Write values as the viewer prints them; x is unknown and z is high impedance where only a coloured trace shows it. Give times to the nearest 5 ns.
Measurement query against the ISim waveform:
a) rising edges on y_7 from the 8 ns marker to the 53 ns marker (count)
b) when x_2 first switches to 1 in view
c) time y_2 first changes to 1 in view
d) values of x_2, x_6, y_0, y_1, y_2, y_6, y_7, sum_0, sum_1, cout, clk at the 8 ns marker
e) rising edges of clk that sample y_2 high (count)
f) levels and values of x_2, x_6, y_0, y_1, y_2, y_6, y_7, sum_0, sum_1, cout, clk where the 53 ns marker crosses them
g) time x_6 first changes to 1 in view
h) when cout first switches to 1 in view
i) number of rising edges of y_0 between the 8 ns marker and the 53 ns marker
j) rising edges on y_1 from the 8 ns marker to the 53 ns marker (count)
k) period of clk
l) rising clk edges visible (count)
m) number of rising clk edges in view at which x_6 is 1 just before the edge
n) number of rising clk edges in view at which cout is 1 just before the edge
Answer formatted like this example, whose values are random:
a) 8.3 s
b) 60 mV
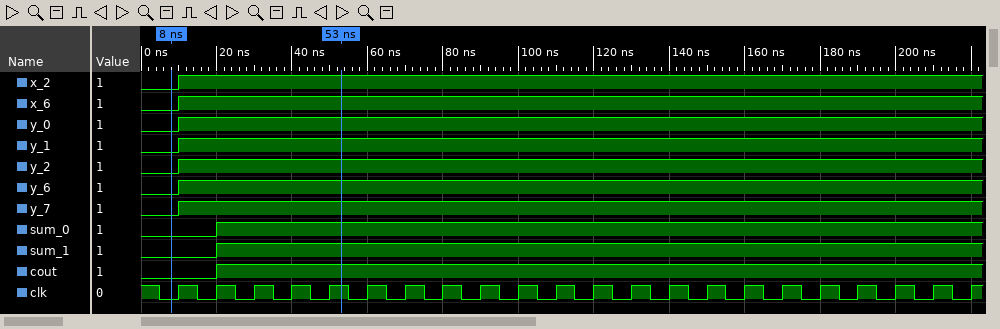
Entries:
a) 1
b) 10 ns
c) 10 ns
d) x_2=0, x_6=0, y_0=0, y_1=0, y_2=0, y_6=0, y_7=0, sum_0=0, sum_1=0, cout=0, clk=0
e) 21
f) x_2=1, x_6=1, y_0=1, y_1=1, y_2=1, y_6=1, y_7=1, sum_0=1, sum_1=1, cout=1, clk=1
g) 10 ns
h) 20 ns
i) 1
j) 1
k) 10 ns
l) 22
m) 21
n) 20
